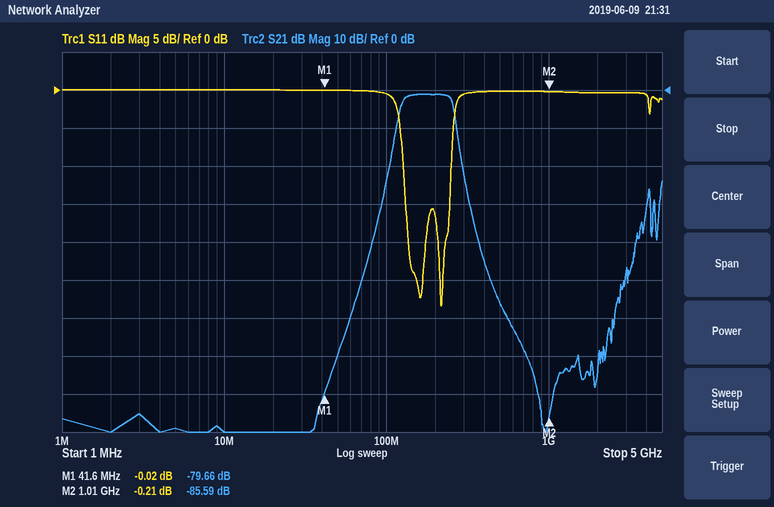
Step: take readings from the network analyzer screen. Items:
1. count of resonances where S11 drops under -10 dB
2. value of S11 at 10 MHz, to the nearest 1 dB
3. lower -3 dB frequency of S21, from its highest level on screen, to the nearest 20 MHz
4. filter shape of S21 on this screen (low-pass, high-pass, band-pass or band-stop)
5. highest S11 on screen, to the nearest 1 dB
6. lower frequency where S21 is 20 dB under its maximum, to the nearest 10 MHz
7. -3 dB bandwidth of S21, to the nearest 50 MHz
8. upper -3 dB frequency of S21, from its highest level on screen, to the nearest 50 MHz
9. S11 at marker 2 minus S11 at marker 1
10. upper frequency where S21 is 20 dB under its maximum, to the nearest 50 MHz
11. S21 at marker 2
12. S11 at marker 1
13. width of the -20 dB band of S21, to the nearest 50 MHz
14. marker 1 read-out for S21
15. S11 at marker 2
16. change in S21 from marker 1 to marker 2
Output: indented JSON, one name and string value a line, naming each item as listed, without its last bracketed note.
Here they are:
{
  "count of resonances where S11 drops under -10 dB": "2",
  "value of S11 at 10 MHz, to the nearest 1 dB": "0 dB",
  "lower -3 dB frequency of S21, from its highest level on screen, to the nearest 20 MHz": "120 MHz",
  "filter shape of S21 on this screen": "band-pass",
  "highest S11 on screen, to the nearest 1 dB": "0 dB",
  "lower frequency where S21 is 20 dB under its maximum, to the nearest 10 MHz": "100 MHz",
  "-3 dB bandwidth of S21, to the nearest 50 MHz": "150 MHz",
  "upper -3 dB frequency of S21, from its highest level on screen, to the nearest 50 MHz": "250 MHz",
  "S11 at marker 2 minus S11 at marker 1": "-0.19 dB",
  "upper frequency where S21 is 20 dB under its maximum, to the nearest 50 MHz": "300 MHz",
  "S21 at marker 2": "-85.59 dB",
  "S11 at marker 1": "-0.02 dB",
  "width of the -20 dB band of S21, to the nearest 50 MHz": "200 MHz",
  "marker 1 read-out for S21": "-79.66 dB",
  "S11 at marker 2": "-0.21 dB",
  "change in S21 from marker 1 to marker 2": "-5.93 dB"
}
